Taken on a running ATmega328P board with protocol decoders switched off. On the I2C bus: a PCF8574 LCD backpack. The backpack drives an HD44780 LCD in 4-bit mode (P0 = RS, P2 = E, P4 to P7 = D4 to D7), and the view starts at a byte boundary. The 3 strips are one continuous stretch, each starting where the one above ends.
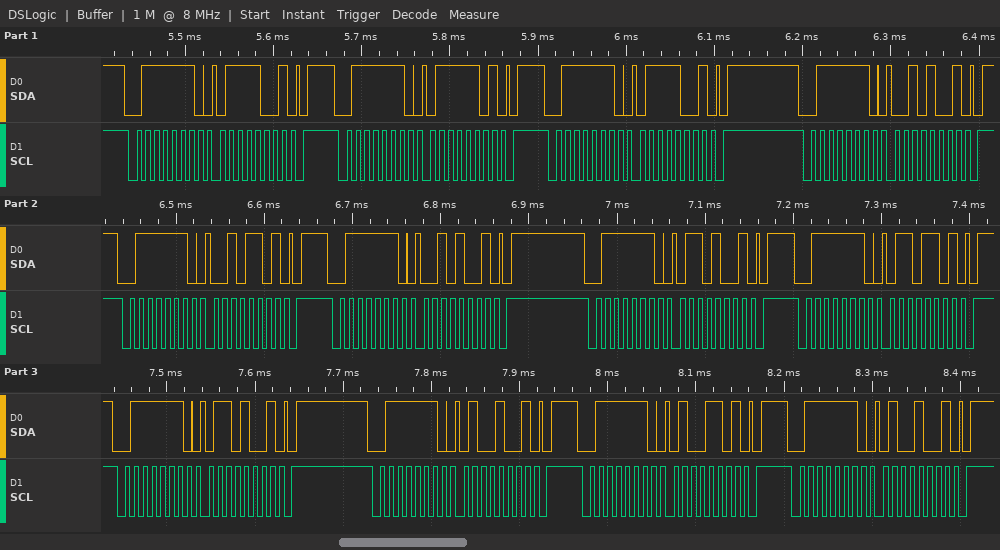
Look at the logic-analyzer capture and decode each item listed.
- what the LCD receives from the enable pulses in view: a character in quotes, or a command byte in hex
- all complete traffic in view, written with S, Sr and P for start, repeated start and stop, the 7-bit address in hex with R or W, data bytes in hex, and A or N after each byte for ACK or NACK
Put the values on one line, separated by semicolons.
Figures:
'r' 'd'; S 3FW A 79 A P S 3FW A 7D A P S 3FW A 79 A P S 3FW A 29 A P S 3FW A 2D A P S 3FW A 29 A P S 3FW A 69 A P S 3FW A 6D A P S 3FW A 69 A P S 3FW A 49 A P S 3FW A 4D A P S 3FW A 49 A P
